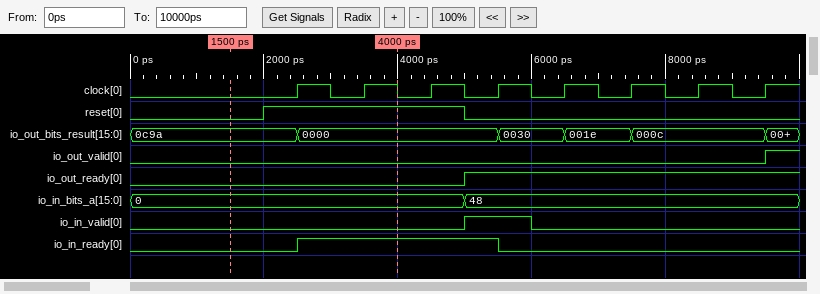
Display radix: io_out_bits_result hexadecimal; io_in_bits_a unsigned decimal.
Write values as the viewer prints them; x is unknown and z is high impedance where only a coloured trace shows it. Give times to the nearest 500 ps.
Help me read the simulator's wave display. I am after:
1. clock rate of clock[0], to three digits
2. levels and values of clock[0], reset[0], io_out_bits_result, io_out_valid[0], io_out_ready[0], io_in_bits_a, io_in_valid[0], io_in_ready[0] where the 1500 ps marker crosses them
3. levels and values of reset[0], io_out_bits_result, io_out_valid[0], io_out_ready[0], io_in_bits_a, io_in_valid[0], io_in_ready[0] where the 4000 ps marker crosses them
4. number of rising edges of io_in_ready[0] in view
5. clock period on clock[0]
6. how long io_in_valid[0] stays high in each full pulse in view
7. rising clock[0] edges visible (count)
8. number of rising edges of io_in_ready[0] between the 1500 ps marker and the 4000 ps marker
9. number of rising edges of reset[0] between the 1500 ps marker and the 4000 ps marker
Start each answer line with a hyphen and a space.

- 1.00 GHz
- clock[0]=0, reset[0]=0, io_out_bits_result=0c9a, io_out_valid[0]=0, io_out_ready[0]=0, io_in_bits_a=0, io_in_valid[0]=0, io_in_ready[0]=0
- reset[0]=1, io_out_bits_result=0000, io_out_valid[0]=0, io_out_ready[0]=0, io_in_bits_a=0, io_in_valid[0]=0, io_in_ready[0]=1
- 1
- 1000 ps
- 1000 ps
- 8
- 1
- 1
